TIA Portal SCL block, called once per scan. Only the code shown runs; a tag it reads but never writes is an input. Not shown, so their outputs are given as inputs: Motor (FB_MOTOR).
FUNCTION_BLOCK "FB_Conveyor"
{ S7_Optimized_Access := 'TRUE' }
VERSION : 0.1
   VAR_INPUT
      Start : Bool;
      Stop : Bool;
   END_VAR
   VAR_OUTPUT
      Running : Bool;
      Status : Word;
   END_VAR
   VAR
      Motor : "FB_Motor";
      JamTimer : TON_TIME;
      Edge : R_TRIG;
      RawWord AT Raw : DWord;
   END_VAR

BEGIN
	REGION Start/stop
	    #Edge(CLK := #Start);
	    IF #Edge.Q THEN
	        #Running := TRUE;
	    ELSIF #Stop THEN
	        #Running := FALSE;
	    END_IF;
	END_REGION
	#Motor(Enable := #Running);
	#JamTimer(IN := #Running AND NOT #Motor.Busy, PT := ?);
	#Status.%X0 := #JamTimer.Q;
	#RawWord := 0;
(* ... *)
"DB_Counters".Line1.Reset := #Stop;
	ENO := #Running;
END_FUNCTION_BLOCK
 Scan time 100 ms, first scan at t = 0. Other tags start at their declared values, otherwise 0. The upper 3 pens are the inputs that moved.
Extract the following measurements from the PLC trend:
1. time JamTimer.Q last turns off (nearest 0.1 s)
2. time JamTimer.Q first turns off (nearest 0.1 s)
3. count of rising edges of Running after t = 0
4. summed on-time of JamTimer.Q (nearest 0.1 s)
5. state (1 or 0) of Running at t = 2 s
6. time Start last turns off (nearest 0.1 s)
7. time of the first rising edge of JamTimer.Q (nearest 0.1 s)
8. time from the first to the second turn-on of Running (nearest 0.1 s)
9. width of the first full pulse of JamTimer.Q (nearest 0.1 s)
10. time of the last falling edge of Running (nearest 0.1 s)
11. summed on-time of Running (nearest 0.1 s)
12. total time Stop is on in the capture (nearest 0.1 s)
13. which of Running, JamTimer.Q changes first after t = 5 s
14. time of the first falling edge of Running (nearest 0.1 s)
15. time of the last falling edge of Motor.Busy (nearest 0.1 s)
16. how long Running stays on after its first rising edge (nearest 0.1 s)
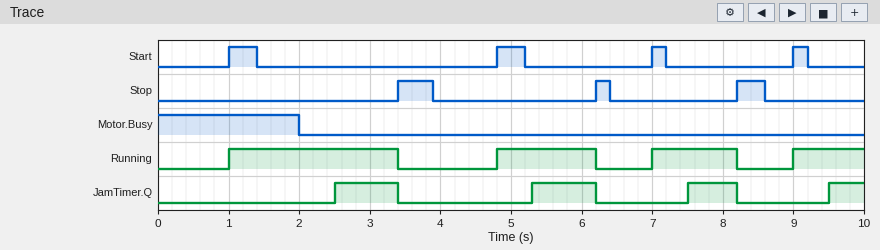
8.2 s
3.4 s
4
3.0 s
1
9.2 s
2.5 s
3.8 s
0.9 s
8.2 s
6.0 s
1.1 s
JamTimer.Q
3.4 s
2.0 s
2.4 s
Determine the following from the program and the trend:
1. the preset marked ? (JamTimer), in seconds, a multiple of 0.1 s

0.5 s
